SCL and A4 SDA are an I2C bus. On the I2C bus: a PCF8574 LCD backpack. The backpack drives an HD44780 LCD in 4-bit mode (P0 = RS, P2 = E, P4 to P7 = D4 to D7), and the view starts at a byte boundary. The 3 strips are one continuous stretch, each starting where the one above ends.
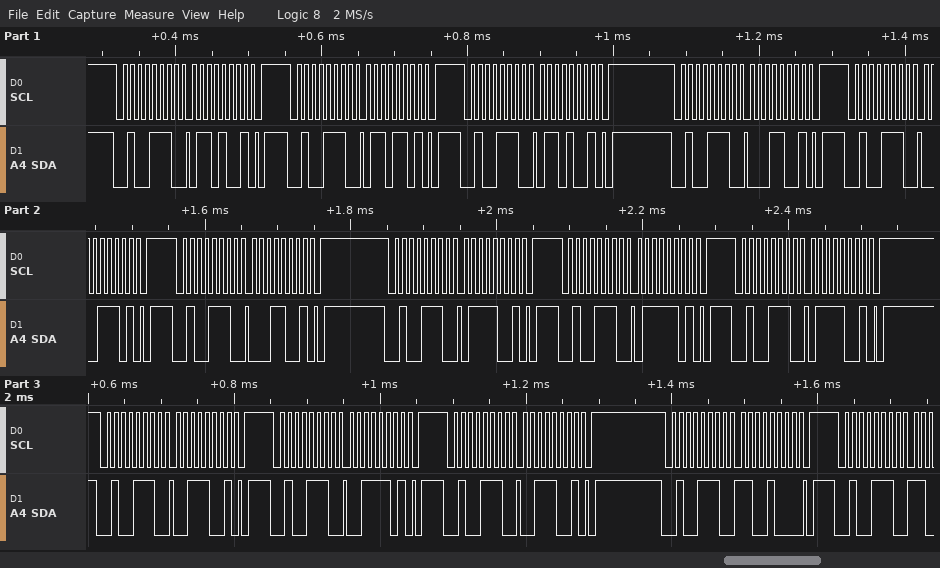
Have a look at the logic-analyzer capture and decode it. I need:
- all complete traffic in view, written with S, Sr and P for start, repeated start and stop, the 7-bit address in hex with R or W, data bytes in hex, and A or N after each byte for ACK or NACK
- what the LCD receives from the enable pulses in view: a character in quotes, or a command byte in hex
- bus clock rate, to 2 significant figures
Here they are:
S 27W A 69 A P S 27W A 6D A P S 27W A 69 A P S 27W A 19 A P S 27W A 1D A P S 27W A 19 A P S 27W A 79 A P S 27W A 7D A P S 27W A 79 A P S 27W A 39 A P S 27W A 3D A P S 27W A 39 A P S 27W A C8 A P S 27W A
'a' 's'
100 kHz
